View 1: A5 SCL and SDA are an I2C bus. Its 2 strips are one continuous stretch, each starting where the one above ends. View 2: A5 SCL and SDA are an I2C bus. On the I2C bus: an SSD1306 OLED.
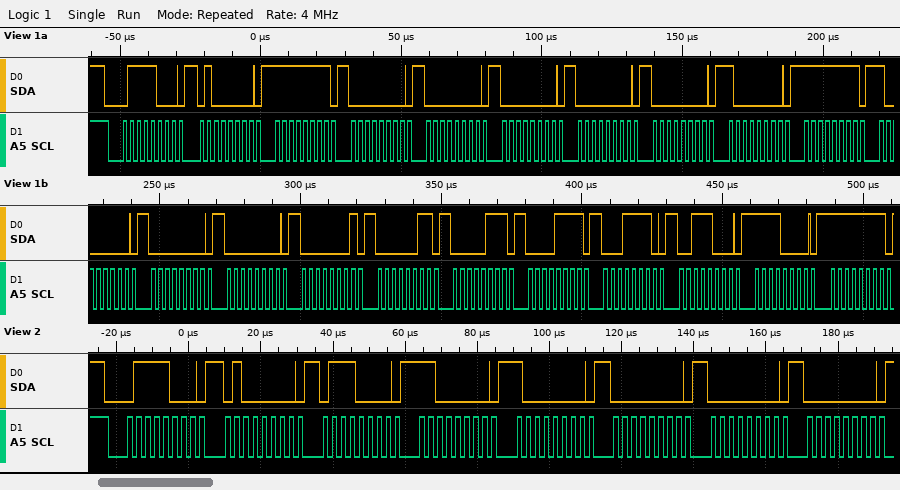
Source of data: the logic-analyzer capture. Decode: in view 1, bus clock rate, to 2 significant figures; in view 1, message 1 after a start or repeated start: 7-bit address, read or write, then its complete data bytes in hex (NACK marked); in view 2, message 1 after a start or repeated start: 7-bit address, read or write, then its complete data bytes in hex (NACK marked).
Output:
400 kHz
0x3C write: 40 FF 00 00 00 00 00 80 FF 80 00 00 01 03 07 0F 1E 38 F0 FF
0x3C write: 40 70 C0 80 00 00 00
